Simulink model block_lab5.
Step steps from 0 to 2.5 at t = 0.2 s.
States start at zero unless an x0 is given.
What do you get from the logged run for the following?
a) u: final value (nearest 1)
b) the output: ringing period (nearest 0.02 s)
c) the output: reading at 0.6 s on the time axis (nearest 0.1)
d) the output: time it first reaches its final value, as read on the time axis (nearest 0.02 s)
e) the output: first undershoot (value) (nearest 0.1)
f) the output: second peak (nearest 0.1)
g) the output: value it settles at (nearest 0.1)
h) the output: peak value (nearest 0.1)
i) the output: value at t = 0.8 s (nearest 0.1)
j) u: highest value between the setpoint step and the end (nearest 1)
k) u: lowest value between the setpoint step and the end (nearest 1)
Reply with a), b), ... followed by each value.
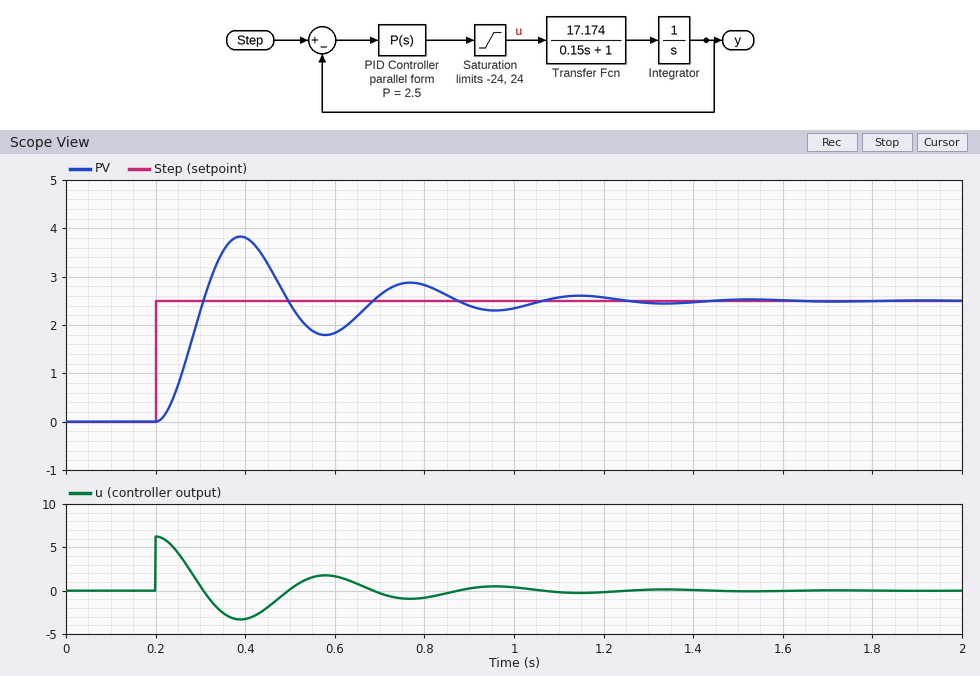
a) 0
b) 0.38 s
c) 1.8
d) 0.30 s
e) 1.8
f) 2.9
g) 2.5
h) 3.8
i) 2.8
j) 6
k) -3
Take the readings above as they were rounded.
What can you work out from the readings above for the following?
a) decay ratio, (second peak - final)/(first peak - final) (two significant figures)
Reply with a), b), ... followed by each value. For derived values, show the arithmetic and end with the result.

a) (2.9 - 2.5) / (3.8 - 2.5) = 0.31
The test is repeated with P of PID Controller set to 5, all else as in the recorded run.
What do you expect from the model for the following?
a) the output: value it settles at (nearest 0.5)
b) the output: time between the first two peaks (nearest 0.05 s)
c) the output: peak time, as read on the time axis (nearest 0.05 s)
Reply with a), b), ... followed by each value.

a) 2.5
b) 0.25 s
c) 0.35 s
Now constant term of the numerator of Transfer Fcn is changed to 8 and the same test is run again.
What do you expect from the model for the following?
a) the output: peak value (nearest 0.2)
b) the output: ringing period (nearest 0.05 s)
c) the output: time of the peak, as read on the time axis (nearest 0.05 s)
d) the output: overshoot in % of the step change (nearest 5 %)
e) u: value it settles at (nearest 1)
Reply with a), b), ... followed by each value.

a) 3.4
b) 0.55 s
c) 0.50 s
d) 40 %
e) 0
